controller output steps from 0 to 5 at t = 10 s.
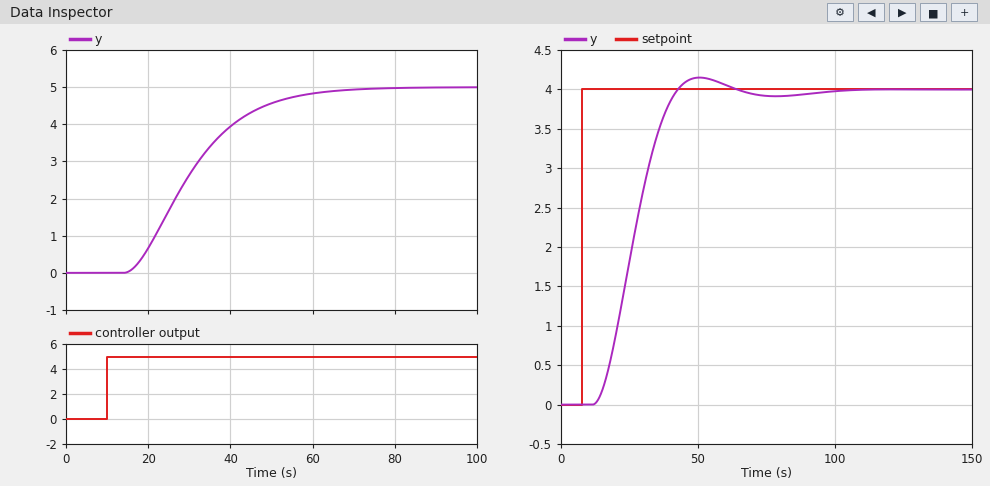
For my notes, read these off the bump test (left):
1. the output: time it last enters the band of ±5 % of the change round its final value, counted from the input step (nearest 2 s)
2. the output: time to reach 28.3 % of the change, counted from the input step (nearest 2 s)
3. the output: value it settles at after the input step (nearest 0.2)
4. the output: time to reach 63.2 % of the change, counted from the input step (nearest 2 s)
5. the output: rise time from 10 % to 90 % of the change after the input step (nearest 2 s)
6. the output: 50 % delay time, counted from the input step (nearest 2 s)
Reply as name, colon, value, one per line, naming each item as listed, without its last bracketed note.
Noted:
the output: time it last enters the band of ±5 % of the change round its final value, counted from the input step: 46 s
the output: time to reach 28.3 % of the change, counted from the input step: 14 s
the output: value it settles at after the input step: 5.0
the output: time to reach 63.2 % of the change, counted from the input step: 24 s
the output: rise time from 10 % to 90 % of the change after the input step: 30 s
the output: 50 % delay time, counted from the input step: 20 s
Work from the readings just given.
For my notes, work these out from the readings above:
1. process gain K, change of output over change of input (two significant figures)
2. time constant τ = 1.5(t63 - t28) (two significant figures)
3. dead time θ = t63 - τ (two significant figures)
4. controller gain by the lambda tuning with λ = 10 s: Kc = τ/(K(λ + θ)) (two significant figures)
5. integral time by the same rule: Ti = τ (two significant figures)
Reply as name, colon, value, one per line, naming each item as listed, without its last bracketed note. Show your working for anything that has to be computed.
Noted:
process gain K, change of output over change of input: (5 - 0) / 5 = 1.0
time constant τ = 1.5(t63 - t28): 1.5 × (24 - 14) = 15 s
dead time θ = t63 - τ: 24 - 15 = 9.0 s
controller gain by the lambda tuning with λ = 10 s: Kc = τ/(K(λ + θ)): 15 / (1 × (10 + 9)) = 0.79
integral time by the same rule: Ti = τ: 15 s
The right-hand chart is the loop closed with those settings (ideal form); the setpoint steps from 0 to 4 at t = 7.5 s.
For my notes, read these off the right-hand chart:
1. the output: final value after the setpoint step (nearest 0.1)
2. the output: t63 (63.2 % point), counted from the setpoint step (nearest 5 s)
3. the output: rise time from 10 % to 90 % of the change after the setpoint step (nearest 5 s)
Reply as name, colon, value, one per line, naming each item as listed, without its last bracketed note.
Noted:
the output: final value after the setpoint step: 4.0
the output: t63 (63.2 % point), counted from the setpoint step: 20 s
the output: rise time from 10 % to 90 % of the change after the setpoint step: 20 s
